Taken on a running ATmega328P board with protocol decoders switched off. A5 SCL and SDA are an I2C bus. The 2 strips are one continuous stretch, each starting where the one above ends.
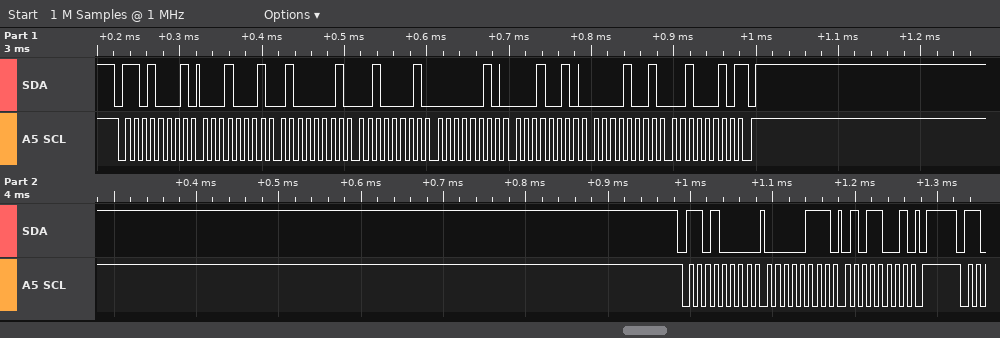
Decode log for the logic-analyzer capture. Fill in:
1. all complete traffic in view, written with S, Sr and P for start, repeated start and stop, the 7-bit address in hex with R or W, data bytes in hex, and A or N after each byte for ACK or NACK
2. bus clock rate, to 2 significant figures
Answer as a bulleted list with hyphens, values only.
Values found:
- S 68R A 11 A 41 A 21 A 02 A 12 A 09 A 22 N P S 68W A 07 A 59 A P
- 100 kHz
